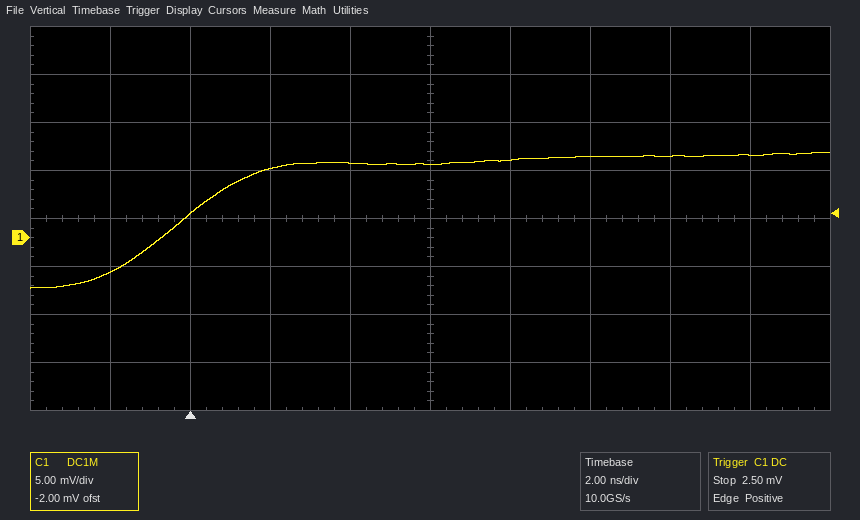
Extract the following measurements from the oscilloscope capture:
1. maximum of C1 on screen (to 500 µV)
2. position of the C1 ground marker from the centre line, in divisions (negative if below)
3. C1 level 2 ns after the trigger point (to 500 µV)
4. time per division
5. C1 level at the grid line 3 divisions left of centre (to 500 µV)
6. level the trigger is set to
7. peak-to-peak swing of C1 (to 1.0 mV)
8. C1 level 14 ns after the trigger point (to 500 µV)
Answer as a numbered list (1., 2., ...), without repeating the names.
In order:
1. 9.0 mV
2. -0.4 div
3. 7.0 mV
4. 2 ns
5. 2.5 mV
6. 2.50 mV
7. 14.0 mV
8. 8.5 mV
